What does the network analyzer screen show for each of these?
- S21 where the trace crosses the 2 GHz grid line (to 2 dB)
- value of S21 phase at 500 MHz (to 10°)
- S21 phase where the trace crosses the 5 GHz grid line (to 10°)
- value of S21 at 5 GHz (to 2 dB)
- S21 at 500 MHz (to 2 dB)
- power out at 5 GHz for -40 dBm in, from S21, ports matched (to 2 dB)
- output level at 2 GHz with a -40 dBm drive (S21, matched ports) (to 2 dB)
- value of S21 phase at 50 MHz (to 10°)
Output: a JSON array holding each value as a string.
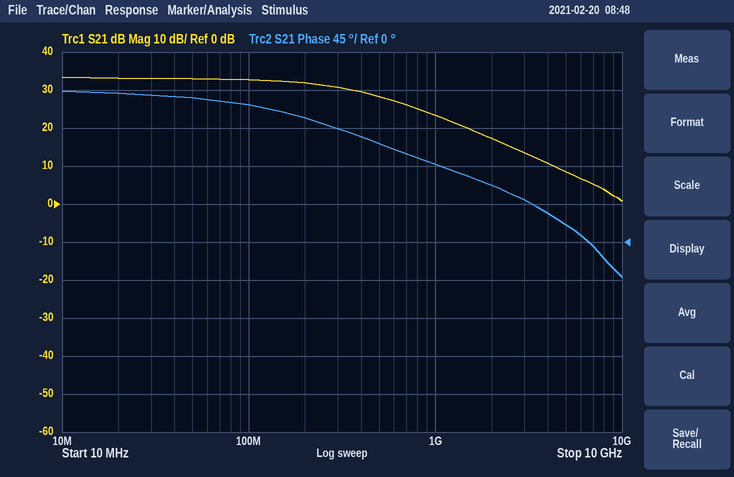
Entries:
["18 dB", "120°", "20°", "8 dB", "28 dB", "-32 dBm", "-22 dBm", "170°"]
